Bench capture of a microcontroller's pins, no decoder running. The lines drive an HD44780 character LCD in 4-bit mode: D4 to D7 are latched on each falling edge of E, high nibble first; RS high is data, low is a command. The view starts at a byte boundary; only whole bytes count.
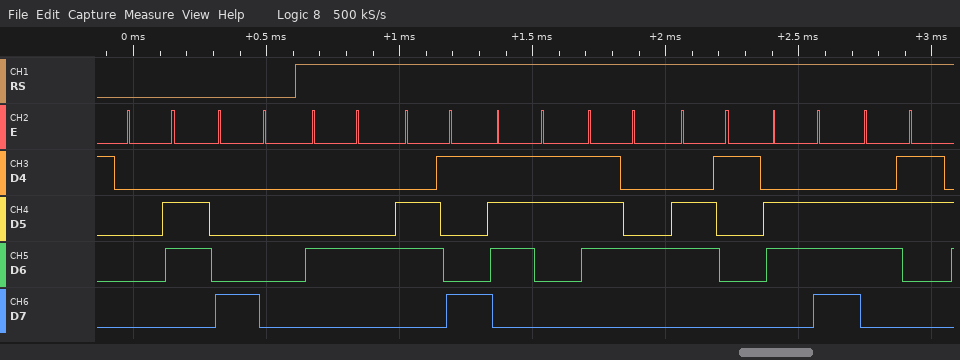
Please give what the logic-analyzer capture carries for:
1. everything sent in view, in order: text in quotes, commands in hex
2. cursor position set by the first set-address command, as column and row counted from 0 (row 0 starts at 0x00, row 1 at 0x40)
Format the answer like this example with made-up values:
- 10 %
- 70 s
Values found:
- 0x06 0x80 "Distanc"
- column 0, row 0
